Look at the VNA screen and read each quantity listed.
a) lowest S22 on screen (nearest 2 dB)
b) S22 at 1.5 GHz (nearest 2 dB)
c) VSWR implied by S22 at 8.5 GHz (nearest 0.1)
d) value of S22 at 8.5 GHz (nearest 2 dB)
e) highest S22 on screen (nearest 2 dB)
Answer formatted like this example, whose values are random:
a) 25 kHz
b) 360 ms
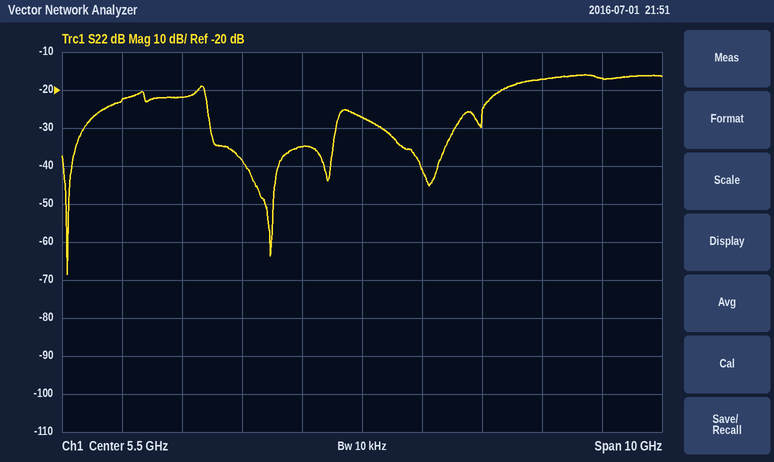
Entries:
a) -68 dB
b) -22 dB
c) 1.3
d) -18 dB
e) -16 dB
